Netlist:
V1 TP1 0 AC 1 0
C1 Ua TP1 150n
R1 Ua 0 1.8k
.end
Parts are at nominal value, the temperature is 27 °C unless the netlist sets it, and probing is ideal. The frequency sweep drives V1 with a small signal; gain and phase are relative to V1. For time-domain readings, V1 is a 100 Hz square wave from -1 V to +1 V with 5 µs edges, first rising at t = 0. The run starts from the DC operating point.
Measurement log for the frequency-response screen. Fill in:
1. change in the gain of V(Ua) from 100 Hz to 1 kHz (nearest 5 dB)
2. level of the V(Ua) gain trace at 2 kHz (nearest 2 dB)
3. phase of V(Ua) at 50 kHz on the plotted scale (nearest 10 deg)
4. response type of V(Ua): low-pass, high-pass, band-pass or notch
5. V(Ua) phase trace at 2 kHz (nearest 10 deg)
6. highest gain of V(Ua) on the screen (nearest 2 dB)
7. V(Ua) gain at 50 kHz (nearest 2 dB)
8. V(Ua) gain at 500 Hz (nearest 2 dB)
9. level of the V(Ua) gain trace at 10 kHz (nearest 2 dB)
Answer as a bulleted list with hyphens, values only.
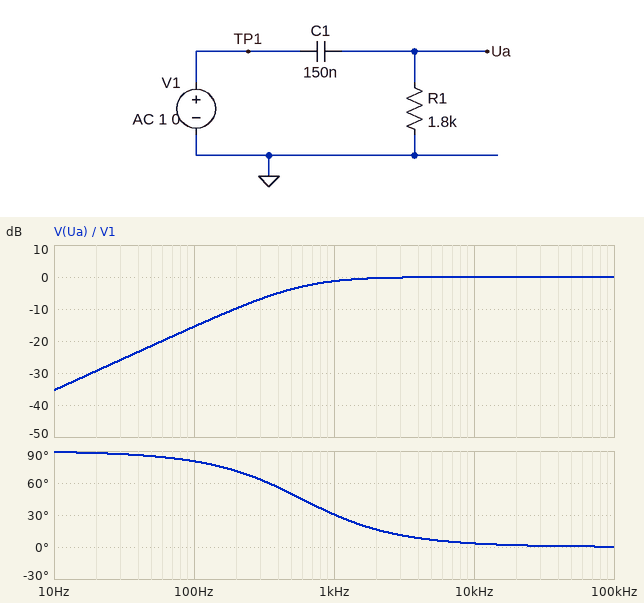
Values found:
- 15 dB
- 0 dB
- 0 deg
- high-pass
- 20 deg
- 0 dB
- 0 dB
- -4 dB
- 0 dB
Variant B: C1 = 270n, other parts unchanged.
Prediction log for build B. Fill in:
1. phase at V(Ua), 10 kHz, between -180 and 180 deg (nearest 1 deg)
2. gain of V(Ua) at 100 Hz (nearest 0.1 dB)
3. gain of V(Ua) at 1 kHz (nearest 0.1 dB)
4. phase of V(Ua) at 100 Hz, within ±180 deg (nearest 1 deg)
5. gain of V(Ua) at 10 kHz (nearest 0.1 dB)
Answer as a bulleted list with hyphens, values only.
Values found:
- 2 deg
- -10.7 dB
- -0.4 dB
- 73 deg
- 0 dB
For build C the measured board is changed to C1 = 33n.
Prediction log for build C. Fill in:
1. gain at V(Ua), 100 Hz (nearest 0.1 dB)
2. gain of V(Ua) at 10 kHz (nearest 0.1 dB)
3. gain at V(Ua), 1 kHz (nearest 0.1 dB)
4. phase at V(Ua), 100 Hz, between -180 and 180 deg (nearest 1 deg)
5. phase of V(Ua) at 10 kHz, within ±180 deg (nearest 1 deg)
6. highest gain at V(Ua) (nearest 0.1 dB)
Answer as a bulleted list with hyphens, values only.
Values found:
- -28.6 dB
- -0.3 dB
- -9.1 dB
- 88 deg
- 15 deg
- 0 dB
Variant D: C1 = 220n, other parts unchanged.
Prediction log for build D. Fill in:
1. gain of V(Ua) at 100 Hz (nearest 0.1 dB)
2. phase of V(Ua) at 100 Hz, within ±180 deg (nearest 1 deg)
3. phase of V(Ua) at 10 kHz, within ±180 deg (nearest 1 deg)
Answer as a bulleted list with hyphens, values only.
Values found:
- -12.3 dB
- 76 deg
- 2 deg
